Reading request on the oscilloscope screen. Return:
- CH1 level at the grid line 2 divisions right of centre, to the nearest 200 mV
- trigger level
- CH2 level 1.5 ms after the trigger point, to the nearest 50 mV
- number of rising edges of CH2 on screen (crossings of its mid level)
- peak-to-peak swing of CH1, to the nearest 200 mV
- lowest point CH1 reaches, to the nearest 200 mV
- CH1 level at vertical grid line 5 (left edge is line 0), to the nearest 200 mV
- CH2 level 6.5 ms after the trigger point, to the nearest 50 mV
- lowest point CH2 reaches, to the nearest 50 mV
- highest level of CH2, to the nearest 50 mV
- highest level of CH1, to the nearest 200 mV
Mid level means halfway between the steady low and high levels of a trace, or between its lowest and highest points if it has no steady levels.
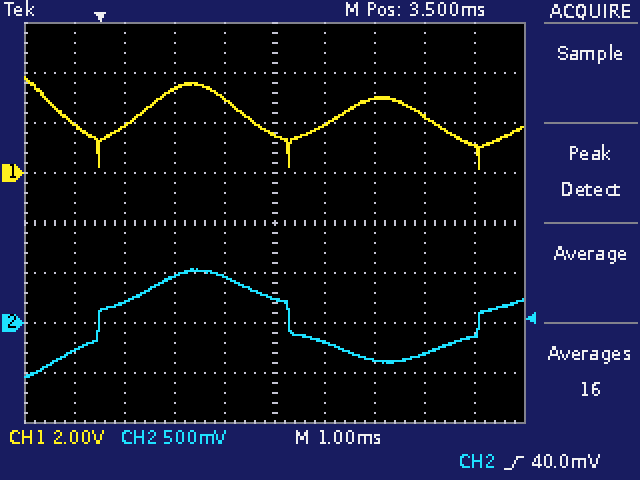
3.0 V
40.0 mV
450 mV
2
3.6 V
200 mV
1.6 V
-300 mV
-550 mV
550 mV
3.8 V
